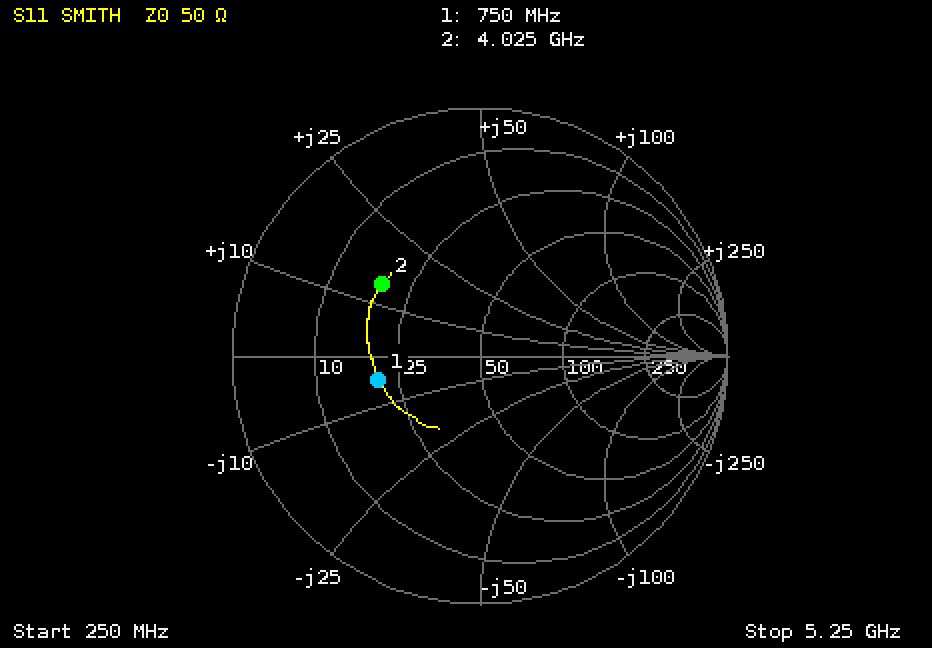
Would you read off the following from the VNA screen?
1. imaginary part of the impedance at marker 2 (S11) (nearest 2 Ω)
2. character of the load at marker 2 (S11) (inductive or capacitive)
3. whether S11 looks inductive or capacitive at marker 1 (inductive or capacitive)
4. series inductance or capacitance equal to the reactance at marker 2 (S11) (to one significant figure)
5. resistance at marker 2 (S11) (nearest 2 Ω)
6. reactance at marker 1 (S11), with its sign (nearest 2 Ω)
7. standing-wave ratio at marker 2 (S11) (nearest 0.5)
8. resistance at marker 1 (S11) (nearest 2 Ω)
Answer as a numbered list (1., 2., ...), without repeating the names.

1. +14 Ω
2. inductive
3. capacitive
4. 600 pH
5. 18 Ω
6. -4 Ω
7. 3.0
8. 20 Ω
